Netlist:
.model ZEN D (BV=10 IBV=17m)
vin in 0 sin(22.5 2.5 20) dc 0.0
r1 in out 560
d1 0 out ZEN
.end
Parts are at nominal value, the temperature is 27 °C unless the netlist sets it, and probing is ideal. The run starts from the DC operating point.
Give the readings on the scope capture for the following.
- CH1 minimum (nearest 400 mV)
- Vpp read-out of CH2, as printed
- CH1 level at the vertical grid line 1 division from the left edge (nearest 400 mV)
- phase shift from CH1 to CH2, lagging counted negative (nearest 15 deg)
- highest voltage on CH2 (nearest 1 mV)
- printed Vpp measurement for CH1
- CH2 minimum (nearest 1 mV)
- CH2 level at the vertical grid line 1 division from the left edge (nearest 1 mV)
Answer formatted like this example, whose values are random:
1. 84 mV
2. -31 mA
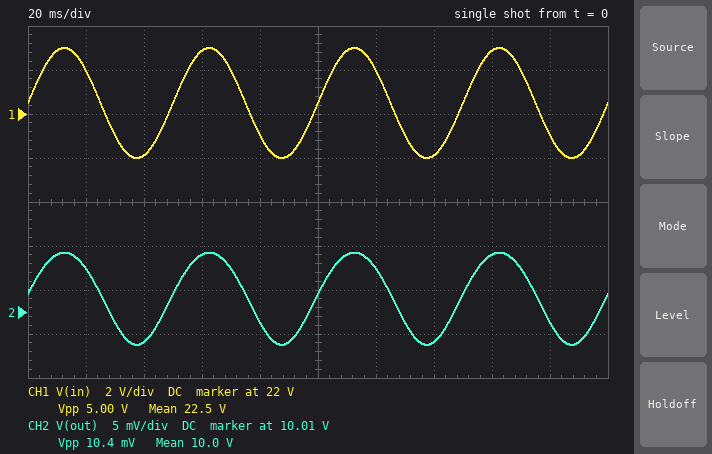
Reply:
1. 20.0 V
2. 10.4 mV
3. 24.0 V
4. 0 deg
5. 10.012 V
6. 5.00 V
7. 10.001 V
8. 10.010 V
